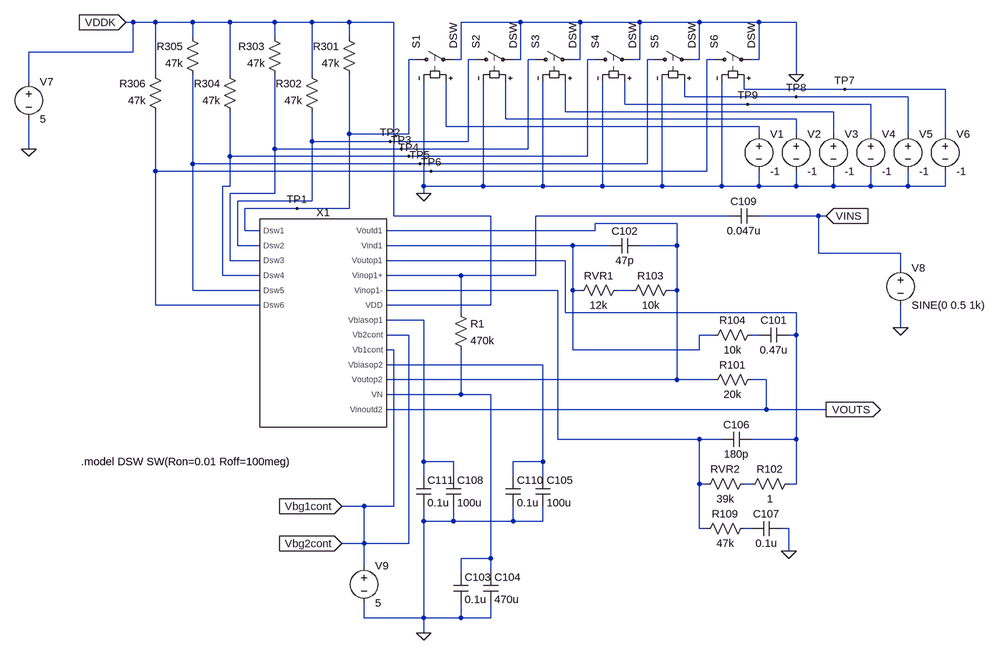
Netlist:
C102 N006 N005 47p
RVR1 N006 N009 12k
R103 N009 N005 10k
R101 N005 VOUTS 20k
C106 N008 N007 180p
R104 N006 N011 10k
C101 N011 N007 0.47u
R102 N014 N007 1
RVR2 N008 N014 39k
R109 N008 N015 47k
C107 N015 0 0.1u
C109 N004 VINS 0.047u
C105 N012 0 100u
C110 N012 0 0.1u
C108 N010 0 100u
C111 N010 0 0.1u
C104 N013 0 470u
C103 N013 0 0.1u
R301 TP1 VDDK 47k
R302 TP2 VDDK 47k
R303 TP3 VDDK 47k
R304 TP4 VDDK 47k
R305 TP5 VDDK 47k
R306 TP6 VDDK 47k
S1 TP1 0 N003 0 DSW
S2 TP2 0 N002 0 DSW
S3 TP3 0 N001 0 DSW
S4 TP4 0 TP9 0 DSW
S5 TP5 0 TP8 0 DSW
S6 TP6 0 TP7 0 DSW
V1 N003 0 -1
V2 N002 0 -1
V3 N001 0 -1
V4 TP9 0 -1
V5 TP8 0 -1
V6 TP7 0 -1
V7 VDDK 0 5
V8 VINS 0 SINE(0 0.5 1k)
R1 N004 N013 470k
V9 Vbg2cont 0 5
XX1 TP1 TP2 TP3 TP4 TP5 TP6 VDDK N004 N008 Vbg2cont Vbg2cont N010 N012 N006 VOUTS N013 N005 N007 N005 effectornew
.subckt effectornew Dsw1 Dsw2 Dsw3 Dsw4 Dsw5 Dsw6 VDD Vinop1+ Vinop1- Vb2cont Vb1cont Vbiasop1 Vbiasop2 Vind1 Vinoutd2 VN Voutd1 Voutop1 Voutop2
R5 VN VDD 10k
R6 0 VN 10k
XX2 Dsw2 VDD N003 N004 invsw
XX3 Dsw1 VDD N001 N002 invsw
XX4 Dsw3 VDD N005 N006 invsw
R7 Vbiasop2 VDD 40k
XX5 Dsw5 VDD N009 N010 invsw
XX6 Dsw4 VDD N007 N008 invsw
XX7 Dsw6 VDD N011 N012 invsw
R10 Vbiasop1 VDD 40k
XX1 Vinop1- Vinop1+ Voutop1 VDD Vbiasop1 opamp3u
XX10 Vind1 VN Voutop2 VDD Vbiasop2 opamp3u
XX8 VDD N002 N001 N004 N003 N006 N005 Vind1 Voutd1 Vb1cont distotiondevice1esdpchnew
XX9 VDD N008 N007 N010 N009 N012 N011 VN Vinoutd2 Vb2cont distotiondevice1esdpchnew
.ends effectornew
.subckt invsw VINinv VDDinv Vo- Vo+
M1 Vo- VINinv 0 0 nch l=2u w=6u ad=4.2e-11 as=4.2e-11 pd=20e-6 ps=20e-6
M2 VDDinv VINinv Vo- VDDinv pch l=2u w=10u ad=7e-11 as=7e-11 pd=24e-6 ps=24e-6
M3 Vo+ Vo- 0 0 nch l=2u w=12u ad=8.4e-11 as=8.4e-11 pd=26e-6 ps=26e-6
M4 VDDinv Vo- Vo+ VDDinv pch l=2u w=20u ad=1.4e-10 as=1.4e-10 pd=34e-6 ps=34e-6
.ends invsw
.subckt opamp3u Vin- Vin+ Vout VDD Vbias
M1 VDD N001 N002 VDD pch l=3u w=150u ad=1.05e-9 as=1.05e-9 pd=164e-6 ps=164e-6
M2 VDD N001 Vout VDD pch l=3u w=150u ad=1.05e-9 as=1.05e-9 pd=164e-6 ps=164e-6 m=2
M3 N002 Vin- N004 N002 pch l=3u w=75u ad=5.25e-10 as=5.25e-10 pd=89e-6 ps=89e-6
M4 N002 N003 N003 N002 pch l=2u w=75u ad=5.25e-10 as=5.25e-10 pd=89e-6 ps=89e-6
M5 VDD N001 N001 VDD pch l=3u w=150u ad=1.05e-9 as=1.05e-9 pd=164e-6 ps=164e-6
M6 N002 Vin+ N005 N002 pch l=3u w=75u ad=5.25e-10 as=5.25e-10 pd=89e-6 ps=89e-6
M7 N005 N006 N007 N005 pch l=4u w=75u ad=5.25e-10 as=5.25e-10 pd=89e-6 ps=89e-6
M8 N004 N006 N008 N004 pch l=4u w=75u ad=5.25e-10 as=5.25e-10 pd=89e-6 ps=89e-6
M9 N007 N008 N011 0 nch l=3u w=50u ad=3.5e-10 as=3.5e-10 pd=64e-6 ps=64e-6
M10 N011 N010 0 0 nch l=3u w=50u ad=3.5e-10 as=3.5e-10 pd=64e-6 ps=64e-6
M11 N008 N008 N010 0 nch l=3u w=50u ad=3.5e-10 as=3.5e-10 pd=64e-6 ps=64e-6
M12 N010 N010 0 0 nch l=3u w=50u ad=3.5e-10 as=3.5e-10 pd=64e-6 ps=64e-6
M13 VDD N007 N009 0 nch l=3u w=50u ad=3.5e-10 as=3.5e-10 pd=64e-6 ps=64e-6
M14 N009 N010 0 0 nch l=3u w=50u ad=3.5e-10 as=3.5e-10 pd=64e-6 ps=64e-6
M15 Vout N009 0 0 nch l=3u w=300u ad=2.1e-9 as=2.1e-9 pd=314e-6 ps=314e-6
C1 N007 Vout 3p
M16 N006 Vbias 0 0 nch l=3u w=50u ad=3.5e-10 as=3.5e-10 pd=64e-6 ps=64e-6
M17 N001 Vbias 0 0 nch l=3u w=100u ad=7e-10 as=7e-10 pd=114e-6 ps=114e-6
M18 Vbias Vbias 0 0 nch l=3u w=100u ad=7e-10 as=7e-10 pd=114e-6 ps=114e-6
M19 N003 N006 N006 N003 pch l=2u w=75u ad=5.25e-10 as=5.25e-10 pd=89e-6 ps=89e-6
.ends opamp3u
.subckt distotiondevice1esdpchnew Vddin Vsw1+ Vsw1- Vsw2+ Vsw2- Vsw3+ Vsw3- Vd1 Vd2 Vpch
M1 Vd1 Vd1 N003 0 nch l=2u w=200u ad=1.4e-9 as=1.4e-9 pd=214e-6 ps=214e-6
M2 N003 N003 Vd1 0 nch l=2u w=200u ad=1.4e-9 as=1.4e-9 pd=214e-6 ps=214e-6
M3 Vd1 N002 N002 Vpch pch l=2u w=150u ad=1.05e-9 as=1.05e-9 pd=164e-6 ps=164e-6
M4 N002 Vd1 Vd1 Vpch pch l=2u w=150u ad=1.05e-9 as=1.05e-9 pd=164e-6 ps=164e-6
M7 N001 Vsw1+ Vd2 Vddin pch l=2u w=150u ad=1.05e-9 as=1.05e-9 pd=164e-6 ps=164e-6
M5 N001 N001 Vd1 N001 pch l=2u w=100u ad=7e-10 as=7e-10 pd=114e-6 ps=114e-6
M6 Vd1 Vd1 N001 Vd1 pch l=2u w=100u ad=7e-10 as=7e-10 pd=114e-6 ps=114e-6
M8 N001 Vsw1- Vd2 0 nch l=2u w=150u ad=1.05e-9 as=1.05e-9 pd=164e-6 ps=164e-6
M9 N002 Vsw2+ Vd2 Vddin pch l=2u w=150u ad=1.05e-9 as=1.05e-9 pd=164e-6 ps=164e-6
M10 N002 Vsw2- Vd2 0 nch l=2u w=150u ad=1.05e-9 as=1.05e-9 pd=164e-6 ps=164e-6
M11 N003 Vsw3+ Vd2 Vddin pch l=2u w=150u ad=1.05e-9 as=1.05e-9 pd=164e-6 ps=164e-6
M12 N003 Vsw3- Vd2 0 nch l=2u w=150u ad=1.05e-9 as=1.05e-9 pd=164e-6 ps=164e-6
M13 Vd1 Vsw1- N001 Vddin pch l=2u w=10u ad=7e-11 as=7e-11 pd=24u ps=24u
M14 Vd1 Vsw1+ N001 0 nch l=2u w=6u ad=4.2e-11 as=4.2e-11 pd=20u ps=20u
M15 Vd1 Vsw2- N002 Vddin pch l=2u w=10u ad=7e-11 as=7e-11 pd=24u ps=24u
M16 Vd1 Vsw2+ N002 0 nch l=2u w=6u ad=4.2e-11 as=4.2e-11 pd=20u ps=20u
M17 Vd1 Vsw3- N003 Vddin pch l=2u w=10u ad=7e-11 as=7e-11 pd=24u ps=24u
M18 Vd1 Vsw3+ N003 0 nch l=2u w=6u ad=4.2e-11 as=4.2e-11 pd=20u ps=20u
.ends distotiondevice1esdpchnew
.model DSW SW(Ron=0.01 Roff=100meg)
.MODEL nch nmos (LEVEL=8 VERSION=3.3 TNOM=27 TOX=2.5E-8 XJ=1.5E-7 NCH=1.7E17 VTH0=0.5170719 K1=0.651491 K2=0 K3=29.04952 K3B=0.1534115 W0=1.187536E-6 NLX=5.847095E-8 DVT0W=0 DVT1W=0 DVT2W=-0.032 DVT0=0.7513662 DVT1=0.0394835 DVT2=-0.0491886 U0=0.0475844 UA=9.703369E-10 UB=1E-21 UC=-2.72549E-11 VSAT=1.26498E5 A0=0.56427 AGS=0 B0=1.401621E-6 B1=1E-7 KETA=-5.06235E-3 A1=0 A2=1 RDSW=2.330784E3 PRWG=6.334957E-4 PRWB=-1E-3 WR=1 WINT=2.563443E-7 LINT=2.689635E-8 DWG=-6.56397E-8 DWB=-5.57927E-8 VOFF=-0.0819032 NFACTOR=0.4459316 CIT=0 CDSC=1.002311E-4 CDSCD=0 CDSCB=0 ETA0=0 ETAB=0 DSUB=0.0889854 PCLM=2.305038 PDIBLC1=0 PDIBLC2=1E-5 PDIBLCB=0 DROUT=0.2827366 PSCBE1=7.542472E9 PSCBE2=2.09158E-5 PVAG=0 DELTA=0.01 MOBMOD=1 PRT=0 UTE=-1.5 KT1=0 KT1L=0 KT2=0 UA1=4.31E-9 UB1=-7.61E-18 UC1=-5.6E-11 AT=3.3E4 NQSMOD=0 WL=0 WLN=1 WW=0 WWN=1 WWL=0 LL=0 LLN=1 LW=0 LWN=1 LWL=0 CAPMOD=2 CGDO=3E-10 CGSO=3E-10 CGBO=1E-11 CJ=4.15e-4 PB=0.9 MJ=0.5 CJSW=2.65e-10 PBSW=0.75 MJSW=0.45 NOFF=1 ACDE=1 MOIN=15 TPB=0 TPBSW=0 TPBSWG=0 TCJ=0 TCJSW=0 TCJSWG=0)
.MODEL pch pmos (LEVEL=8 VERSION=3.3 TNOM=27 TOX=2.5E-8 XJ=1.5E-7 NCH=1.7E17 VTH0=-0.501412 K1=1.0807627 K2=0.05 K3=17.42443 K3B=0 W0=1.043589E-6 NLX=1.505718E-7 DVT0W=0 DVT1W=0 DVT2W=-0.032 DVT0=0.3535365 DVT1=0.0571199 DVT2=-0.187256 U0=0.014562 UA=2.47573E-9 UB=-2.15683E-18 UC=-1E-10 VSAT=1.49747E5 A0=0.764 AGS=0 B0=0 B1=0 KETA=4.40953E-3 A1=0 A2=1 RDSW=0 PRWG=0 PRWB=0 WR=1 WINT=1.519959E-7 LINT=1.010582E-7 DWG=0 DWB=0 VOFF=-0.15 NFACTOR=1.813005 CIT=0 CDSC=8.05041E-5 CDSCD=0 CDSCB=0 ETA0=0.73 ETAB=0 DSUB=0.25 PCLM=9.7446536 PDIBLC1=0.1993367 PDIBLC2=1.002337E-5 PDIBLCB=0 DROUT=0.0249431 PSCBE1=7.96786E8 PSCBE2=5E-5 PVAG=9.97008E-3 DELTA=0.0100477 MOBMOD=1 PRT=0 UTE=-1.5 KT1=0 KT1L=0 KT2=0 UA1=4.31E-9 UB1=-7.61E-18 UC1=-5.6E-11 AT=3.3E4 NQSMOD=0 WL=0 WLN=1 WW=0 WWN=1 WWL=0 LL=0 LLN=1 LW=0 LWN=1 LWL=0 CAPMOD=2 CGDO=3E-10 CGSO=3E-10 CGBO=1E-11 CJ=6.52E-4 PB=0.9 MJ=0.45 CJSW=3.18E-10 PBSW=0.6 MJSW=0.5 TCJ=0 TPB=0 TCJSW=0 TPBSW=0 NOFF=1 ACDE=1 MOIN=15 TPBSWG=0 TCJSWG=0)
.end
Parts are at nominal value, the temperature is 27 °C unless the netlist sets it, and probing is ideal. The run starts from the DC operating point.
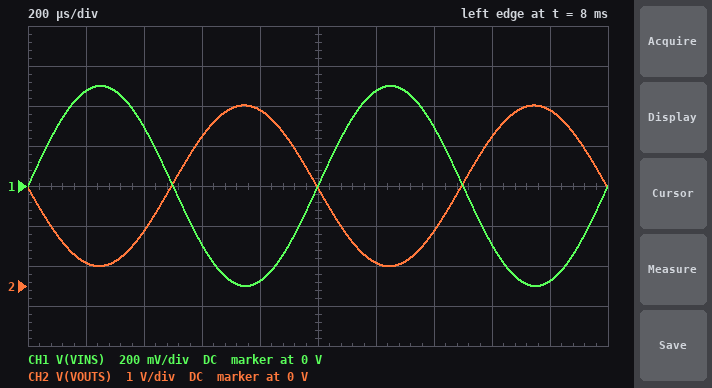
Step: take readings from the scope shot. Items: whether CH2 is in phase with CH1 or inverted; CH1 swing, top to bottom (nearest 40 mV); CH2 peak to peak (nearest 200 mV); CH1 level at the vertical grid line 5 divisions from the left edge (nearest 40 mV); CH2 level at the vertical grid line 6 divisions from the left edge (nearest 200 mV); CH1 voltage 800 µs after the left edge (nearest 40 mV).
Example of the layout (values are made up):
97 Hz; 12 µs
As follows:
inverted; 1.00 V; 4.0 V; 0 V; 600 mV; -480 mV
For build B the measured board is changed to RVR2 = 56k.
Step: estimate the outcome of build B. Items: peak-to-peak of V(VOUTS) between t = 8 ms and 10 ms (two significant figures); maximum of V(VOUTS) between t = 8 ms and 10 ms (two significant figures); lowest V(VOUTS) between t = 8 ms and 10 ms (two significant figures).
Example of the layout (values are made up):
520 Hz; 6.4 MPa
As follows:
4.8 V; 4.9 V; 100 mV
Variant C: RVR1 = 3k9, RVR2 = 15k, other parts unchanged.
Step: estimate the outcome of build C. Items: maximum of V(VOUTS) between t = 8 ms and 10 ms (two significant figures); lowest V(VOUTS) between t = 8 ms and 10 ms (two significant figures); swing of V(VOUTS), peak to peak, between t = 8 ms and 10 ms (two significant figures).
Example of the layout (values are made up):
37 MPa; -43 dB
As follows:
3.4 V; 1.6 V; 1.8 V
